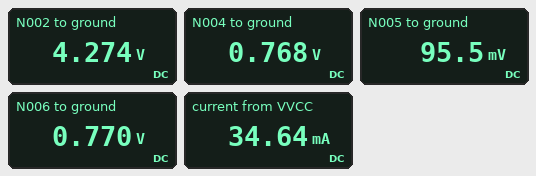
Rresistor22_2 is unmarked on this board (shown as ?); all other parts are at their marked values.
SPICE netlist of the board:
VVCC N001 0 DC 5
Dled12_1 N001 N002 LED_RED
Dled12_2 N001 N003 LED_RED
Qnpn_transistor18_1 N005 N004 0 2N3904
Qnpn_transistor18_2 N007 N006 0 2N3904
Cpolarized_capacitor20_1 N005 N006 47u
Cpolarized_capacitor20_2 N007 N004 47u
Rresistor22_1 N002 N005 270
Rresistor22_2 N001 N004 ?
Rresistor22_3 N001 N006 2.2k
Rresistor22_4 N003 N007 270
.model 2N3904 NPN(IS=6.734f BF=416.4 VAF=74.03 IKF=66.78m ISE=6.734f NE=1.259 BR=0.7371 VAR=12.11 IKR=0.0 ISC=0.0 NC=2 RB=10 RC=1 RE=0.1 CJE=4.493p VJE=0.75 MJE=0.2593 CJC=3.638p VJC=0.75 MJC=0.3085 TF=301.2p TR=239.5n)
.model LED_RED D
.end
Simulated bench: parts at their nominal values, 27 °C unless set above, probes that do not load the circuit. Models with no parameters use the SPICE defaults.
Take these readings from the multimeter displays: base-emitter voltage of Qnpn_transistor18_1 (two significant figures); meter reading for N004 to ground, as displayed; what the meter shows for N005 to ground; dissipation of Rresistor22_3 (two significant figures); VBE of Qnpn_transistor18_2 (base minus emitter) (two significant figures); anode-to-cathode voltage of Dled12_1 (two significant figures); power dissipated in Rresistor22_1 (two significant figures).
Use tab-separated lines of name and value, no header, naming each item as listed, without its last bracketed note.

base-emitter voltage of Qnpn_transistor18_1	770 mV
meter reading for N004 to ground, as displayed	0.768 V
what the meter shows for N005 to ground	95.5 mV
dissipation of Rresistor22_3	8.1 mW
VBE of Qnpn_transistor18_2 (base minus emitter)	770 mV
anode-to-cathode voltage of Dled12_1	730 mV
power dissipated in Rresistor22_1	65 mW
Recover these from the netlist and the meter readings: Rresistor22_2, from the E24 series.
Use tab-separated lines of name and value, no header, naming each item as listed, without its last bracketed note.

Rresistor22_2, from the E24 series	2.4 kΩ
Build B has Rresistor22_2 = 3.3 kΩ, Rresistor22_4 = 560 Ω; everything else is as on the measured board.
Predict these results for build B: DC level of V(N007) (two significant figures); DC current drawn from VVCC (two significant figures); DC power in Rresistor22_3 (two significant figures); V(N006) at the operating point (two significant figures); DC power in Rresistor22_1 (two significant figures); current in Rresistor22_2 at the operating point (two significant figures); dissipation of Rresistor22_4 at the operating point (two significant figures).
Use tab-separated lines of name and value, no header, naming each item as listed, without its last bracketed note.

DC level of V(N007)	67 mV
DC current drawn from VVCC	26 mA
DC power in Rresistor22_3	8.2 mW
V(N006) at the operating point	750 mV
DC power in Rresistor22_1	64 mW
current in Rresistor22_2 at the operating point	1.3 mA
dissipation of Rresistor22_4 at the operating point	32 mW
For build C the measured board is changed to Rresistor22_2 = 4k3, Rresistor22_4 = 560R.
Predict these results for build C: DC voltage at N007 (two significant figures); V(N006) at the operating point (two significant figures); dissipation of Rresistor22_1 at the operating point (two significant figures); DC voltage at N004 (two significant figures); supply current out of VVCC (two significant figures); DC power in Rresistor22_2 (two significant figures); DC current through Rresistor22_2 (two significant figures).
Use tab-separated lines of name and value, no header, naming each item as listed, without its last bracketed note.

DC voltage at N007	67 mV
V(N006) at the operating point	750 mV
dissipation of Rresistor22_1 at the operating point	64 mW
DC voltage at N004	760 mV
supply current out of VVCC	26 mA
DC power in Rresistor22_2	4.2 mW
DC current through Rresistor22_2	990 µA
